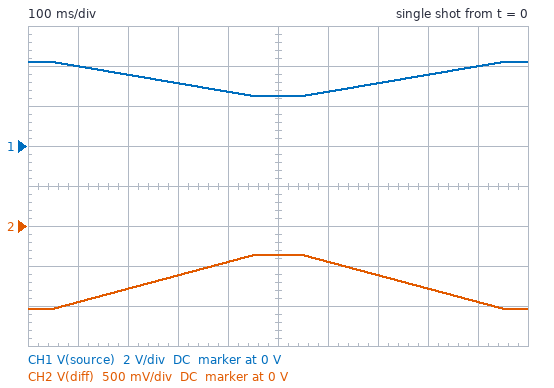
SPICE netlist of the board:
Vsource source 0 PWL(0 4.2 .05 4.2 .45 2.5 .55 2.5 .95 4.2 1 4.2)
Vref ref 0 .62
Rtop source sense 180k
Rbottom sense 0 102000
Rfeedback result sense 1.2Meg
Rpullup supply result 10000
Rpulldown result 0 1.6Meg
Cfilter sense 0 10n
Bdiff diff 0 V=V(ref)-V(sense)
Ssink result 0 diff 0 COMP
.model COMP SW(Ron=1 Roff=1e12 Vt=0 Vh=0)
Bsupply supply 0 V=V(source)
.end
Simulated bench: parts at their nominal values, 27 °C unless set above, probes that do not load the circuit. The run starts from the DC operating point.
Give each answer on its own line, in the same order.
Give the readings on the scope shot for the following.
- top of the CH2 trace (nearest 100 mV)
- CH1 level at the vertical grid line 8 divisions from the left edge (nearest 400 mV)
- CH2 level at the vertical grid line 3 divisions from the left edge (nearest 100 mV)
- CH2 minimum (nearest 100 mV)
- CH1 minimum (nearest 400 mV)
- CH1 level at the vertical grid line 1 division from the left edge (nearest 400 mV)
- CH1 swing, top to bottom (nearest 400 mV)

-400 mV
3.6 V
-600 mV
-1.0 V
2.4 V
4.0 V
1.6 V
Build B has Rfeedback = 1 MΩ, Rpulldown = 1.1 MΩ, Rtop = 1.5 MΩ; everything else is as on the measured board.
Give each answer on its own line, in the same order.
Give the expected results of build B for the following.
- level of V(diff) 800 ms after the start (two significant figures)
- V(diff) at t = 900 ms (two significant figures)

410 mV
390 mV
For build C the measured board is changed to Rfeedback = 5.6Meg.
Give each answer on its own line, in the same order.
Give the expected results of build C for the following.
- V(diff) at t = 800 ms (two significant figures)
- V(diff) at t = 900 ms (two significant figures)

-690 mV
-850 mV
